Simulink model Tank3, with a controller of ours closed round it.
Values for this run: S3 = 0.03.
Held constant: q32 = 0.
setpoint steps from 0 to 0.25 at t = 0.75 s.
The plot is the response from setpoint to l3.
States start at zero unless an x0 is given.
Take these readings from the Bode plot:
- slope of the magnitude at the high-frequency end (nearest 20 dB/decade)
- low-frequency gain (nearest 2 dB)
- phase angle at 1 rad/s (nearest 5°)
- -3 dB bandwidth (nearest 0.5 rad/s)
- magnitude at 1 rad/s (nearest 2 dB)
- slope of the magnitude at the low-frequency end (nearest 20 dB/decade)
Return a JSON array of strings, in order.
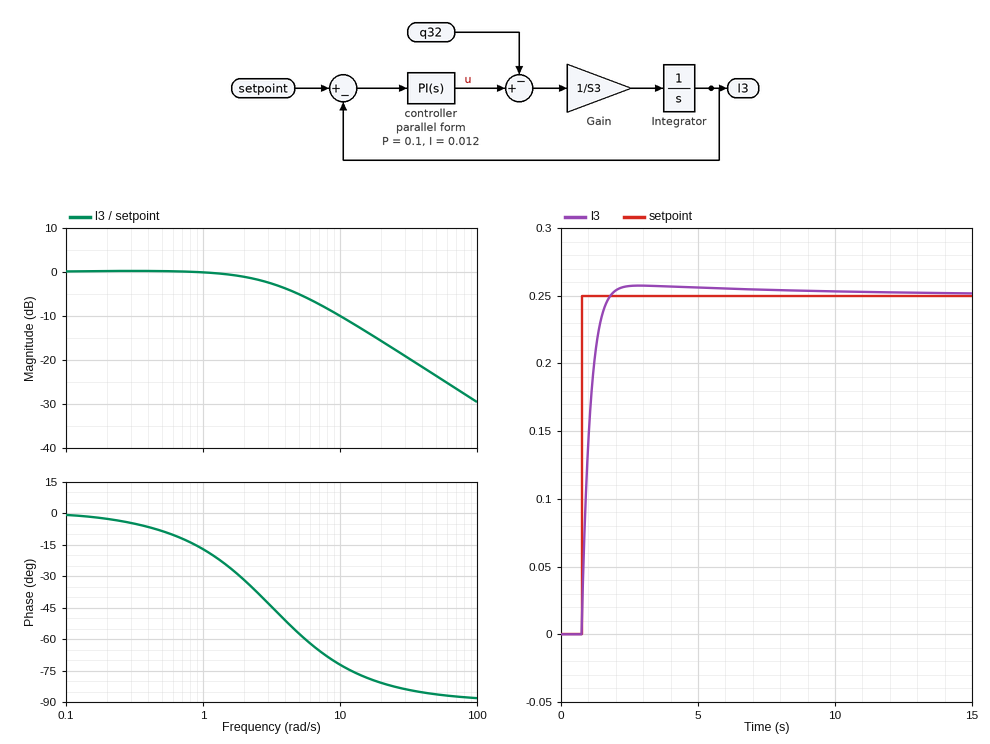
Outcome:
["-20 dB/decade", "0 dB", "-15°", "3.5 rad/s", "0 dB", "0 dB/decade"]
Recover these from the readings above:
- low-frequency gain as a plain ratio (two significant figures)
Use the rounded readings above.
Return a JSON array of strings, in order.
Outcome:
["1.0"]
